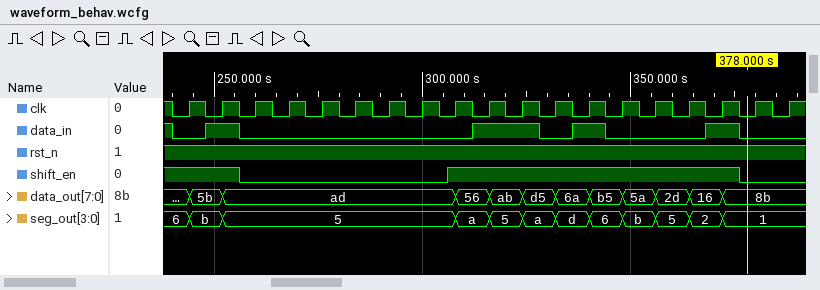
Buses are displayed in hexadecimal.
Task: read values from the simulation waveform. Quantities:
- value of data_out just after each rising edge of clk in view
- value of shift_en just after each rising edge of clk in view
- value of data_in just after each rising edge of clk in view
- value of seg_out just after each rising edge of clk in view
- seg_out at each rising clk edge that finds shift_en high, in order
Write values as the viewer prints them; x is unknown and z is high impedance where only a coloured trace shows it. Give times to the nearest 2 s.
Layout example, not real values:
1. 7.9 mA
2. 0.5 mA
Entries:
1. 5b, ad, ad, ad, ad, ad, ad, ad, 56, ab, d5, 6a, b5, 5a, 2d, 16, 8b, 8b, 8b
2. 1 1 0 0 0 0 0 0 1 1 1 1 1 1 1 1 1 0 0
3. 0 1 0 0 0 0 0 0 0 1 1 0 1 0 0 0 1 0 0
4. b, 5, 5, 5, 5, 5, 5, 5, a, 5, a, d, 6, b, 5, 2, 1, 1, 1
5. 6, b, 5, a, 5, a, d, 6, b, 5, 2
